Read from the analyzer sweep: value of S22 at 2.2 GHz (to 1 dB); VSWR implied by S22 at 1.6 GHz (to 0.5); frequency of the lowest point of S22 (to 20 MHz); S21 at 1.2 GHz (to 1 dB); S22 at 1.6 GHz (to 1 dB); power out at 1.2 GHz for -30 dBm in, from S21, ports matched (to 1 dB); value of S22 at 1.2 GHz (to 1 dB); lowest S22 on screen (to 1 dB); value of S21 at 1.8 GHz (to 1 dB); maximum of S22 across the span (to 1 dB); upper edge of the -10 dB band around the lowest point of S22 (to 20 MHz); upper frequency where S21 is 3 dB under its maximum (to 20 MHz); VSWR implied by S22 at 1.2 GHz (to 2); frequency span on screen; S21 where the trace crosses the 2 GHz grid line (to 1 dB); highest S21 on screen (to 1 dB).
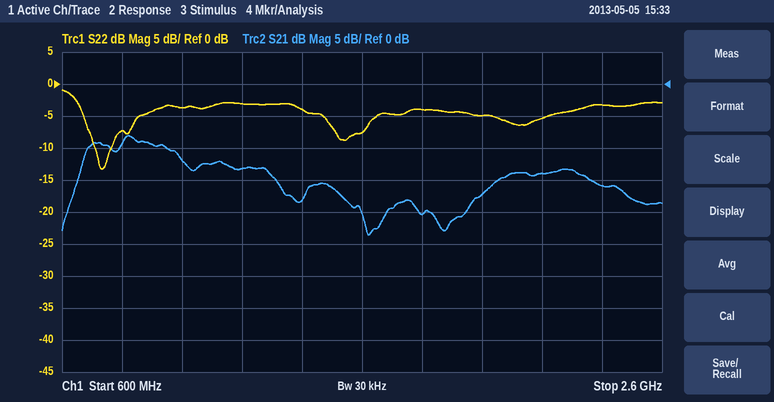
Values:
-5 dB
2.5
740 MHz
-13 dB
-8 dB
-43 dBm
-3 dB
-13 dB
-20 dB
-1 dB
760 MHz
980 MHz
6
2 GHz
-17 dB
-8 dB
